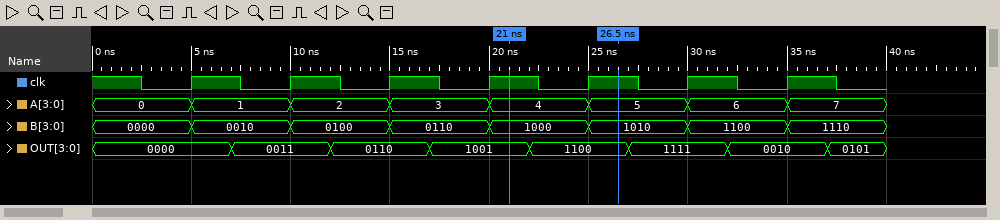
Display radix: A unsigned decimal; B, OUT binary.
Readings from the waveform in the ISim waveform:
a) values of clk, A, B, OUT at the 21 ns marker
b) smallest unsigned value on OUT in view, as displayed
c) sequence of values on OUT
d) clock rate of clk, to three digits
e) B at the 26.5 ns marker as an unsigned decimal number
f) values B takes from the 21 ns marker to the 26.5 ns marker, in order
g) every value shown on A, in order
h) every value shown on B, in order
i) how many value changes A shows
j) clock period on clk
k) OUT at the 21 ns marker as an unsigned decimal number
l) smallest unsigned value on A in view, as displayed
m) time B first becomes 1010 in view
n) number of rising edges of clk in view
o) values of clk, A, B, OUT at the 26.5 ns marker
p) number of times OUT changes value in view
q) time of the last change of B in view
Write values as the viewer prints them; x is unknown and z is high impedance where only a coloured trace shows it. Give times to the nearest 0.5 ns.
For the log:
clk=1, A=4, B=1000, OUT=1001
0000
0000, 0011, 0110, 1001, 1100, 1111, 0010, 0101
200 MHz
10
1000, 1010
0, 1, 2, 3, 4, 5, 6, 7
0000, 0010, 0100, 0110, 1000, 1010, 1100, 1110
7
5 ns
9
0
25 ns
7
clk=1, A=5, B=1010, OUT=1100
7
35 ns
